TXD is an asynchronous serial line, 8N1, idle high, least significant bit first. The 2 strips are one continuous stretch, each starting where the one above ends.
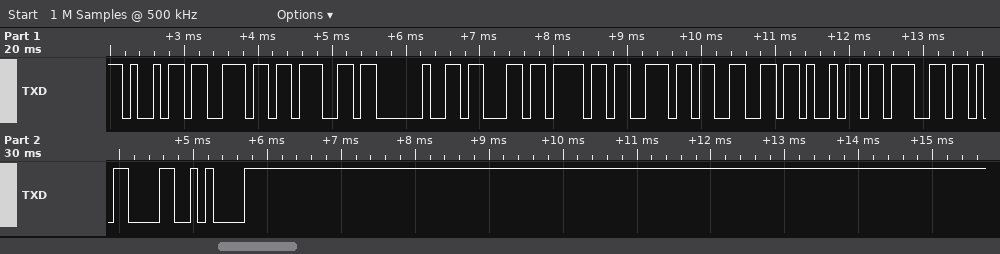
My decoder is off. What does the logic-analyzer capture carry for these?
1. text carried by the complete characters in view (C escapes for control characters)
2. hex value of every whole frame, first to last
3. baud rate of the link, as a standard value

"ing config\r\n"
69 6E 67 20 63 6F 6E 66 69 67 0D 0A
9600 baud
